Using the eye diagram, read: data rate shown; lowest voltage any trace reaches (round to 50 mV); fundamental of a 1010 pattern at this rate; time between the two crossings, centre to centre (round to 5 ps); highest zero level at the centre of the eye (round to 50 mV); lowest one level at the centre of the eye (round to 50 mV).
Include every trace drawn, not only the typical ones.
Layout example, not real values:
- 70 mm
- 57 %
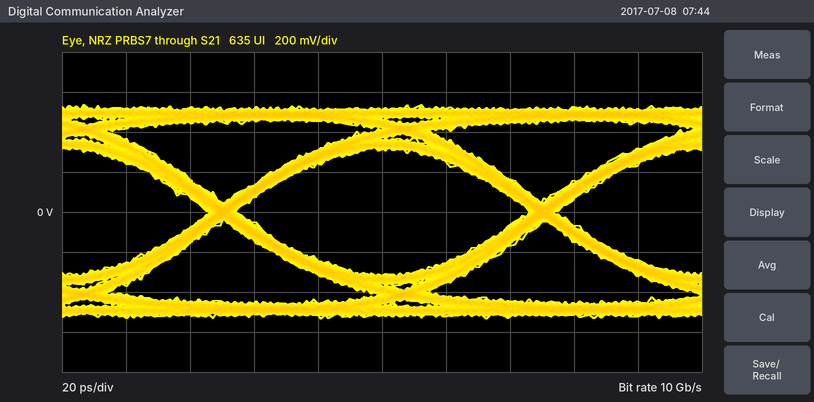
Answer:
- 10 Gb/s
- -550 mV
- 5 GHz
- 100 ps
- -300 mV
- 300 mV
